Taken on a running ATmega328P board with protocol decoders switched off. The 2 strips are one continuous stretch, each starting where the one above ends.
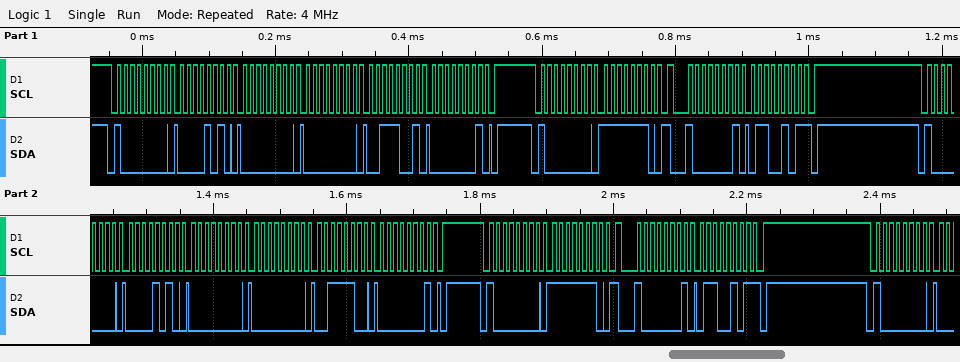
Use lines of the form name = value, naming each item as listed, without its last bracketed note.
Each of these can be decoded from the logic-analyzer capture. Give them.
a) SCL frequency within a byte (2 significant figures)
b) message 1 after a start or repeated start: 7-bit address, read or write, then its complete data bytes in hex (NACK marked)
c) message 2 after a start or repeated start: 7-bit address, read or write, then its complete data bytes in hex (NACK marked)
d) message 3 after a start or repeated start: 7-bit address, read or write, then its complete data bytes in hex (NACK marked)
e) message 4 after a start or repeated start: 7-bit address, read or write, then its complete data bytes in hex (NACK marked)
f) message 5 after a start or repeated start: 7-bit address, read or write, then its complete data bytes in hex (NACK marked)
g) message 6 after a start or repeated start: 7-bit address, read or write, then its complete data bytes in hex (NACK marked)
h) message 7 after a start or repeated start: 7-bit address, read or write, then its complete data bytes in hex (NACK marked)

SCL frequency within a byte = 100 kHz
message 1 after a start or repeated start: 7-bit address, read or write, then its complete data bytes in hex = 0x40 write: 0A 00 00 39 01
message 2 after a start or repeated start: 7-bit address, read or write, then its complete data bytes in hex = 0x40 write: FE
message 3 after a start or repeated start: 7-bit address, read or write, then its complete data bytes in hex = 0x40 read: 65 NACK
message 4 after a start or repeated start: 7-bit address, read or write, then its complete data bytes in hex = 0x40 write: 0A 00 00 3C 01
message 5 after a start or repeated start: 7-bit address, read or write, then its complete data bytes in hex = 0x40 write: FE
message 6 after a start or repeated start: 7-bit address, read or write, then its complete data bytes in hex = 0x40 read: 65 NACK
message 7 after a start or repeated start: 7-bit address, read or write, then its complete data bytes in hex = 0x40 write
